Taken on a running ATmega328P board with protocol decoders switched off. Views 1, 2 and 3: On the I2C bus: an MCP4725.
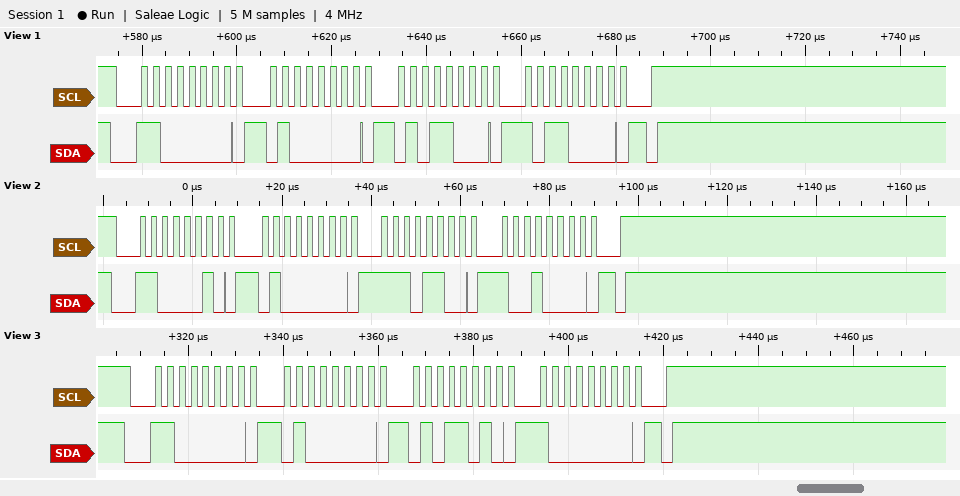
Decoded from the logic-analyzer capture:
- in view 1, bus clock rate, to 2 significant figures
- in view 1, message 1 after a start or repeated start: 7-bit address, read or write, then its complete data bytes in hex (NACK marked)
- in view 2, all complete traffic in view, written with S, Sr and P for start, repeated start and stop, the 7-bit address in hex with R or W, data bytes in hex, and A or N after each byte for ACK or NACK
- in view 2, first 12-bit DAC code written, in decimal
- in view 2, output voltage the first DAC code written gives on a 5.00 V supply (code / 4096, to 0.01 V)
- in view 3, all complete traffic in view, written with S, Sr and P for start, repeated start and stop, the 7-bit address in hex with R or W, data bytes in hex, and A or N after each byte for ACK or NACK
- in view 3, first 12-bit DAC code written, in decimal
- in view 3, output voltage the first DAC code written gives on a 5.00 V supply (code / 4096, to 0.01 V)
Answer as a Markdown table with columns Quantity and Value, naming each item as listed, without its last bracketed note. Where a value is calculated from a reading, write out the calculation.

| Quantity | Value |
|---|---|
| in view 1, bus clock rate, to 2 significant figures | 400 kHz |
| in view 1, message 1 after a start or repeated start: 7-bit address, read or write, then its complete data bytes in hex | 0x60 write: 40 58 B0 |
| in view 2, all complete traffic in view, written with S, Sr and P for start, repeated start and stop, the 7-bit address in hex with R or W, data bytes in hex, and A or N after each byte for ACK or NACK | S 61W A 40 A EC A 90 A P |
| in view 2, first 12-bit DAC code written, in decimal | 3785 |
| in view 2, output voltage the first DAC code written gives on a 5.00 V supply | 3785 / 4096 x 5.00 V = 4.62 V |
| in view 3, all complete traffic in view, written with S, Sr and P for start, repeated start and stop, the 7-bit address in hex with R or W, data bytes in hex, and A or N after each byte for ACK or NACK | S 60W A 40 A 5A A 80 A P |
| in view 3, first 12-bit DAC code written, in decimal | 1448 |
| in view 3, output voltage the first DAC code written gives on a 5.00 V supply | 1448 / 4096 x 5.00 V = 1.77 V |
